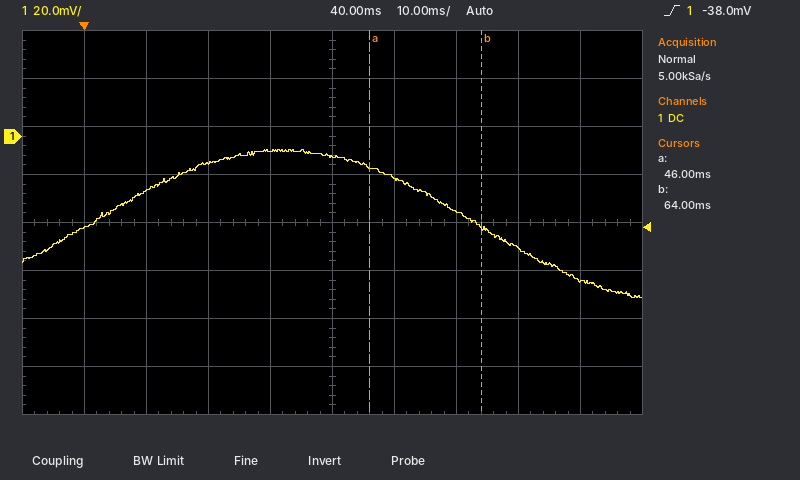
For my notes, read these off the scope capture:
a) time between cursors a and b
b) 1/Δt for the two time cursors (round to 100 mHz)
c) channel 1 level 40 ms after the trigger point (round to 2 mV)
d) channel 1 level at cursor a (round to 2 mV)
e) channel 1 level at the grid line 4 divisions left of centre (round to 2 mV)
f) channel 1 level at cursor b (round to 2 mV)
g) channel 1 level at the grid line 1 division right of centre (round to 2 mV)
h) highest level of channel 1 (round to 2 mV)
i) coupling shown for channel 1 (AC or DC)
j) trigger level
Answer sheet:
18 ms
55.6 Hz
-8 mV
-12 mV
-38 mV
-38 mV
-18 mV
-6 mV
DC
-38.0 mV
